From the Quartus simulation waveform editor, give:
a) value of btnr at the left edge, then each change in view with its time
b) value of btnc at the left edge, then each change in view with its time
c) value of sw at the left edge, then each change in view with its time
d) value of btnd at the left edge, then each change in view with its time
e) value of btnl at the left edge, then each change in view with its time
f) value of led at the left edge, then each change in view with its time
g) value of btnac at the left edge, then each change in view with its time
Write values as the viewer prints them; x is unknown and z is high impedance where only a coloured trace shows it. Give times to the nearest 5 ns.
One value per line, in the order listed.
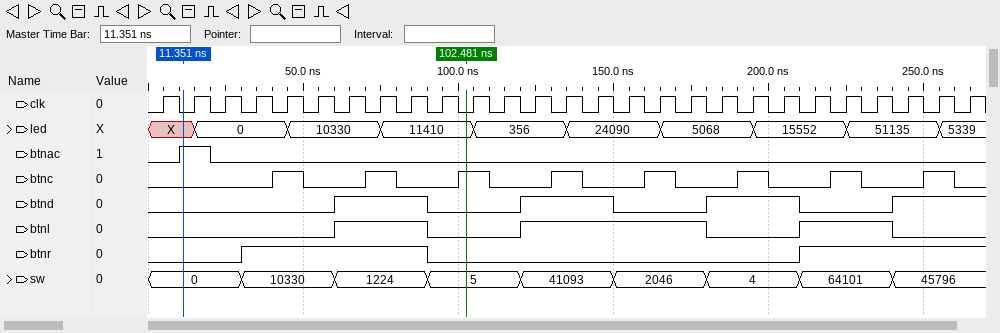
0, 1 at 30 ns, 0 at 90 ns, 1 at 210 ns
0, 1 at 40 ns, 0 at 50 ns, 1 at 70 ns, 0 at 80 ns, 1 at 100 ns, 0 at 110 ns, 1 at 130 ns, 0 at 140 ns, 1 at 160 ns, 0 at 170 ns, 1 at 190 ns, 0 at 200 ns, 1 at 220 ns, 0 at 230 ns, 1 at 250 ns, 0 at 260 ns
0, 10330 at 30 ns, 1224 at 60 ns, 5 at 90 ns, 41093 at 120 ns, 2046 at 150 ns, 4 at 180 ns, 64101 at 210 ns, 45796 at 240 ns
0, 1 at 60 ns, 0 at 90 ns, 1 at 120 ns, 0 at 150 ns, 1 at 180 ns, 0 at 210 ns, 1 at 240 ns
0, 1 at 60 ns, 0 at 90 ns, 1 at 120 ns, 0 at 180 ns, 1 at 210 ns, 0 at 240 ns
X, 0 at 15 ns, 10330 at 45 ns, 11410 at 75 ns, 356 at 105 ns, 24090 at 135 ns, 5068 at 165 ns, 15552 at 195 ns, 51135 at 225 ns, 5339 at 255 ns
0, 1 at 10 ns, 0 at 20 ns
